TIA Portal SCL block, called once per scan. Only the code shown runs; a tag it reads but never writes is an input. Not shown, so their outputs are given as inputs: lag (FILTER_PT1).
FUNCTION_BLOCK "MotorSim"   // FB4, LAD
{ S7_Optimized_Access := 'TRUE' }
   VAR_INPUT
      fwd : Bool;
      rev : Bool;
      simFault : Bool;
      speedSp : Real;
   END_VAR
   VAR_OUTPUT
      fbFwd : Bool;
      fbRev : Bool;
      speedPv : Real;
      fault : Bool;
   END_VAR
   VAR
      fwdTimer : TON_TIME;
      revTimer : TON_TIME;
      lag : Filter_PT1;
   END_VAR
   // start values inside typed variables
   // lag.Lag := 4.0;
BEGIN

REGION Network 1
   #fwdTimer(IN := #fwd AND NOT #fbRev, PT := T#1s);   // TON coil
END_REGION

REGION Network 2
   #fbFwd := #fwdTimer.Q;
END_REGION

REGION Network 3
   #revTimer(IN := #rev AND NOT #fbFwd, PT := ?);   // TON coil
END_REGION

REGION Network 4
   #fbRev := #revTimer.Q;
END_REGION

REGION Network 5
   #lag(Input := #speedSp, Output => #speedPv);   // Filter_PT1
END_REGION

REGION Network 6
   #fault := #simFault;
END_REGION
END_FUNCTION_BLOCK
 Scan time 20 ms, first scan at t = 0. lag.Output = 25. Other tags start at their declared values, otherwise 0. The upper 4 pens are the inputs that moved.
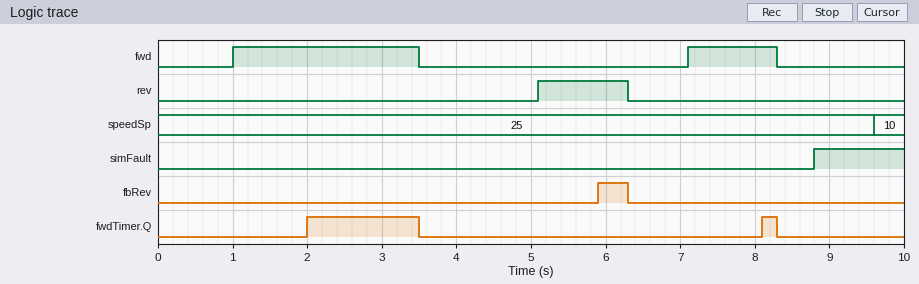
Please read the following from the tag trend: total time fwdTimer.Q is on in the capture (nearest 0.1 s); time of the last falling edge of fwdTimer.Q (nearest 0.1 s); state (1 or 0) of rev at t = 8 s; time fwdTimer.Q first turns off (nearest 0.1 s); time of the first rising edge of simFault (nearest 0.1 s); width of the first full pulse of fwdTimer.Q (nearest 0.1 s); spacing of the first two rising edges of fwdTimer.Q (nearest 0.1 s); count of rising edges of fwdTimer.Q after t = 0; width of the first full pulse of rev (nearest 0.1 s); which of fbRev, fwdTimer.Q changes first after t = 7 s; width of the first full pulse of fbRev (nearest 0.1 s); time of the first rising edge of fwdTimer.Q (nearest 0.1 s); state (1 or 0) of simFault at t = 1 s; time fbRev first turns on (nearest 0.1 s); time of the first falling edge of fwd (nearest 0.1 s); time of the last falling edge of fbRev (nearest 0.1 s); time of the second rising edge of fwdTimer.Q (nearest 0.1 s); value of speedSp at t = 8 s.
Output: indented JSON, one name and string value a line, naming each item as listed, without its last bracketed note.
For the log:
{
  "total time fwdTimer.Q is on in the capture": "1.7 s",
  "time of the last falling edge of fwdTimer.Q": "8.3 s",
  "state (1 or 0) of rev at t = 8 s": "0",
  "time fwdTimer.Q first turns off": "3.5 s",
  "time of the first rising edge of simFault": "8.8 s",
  "width of the first full pulse of fwdTimer.Q": "1.5 s",
  "spacing of the first two rising edges of fwdTimer.Q": "6.1 s",
  "count of rising edges of fwdTimer.Q after t = 0": "2",
  "width of the first full pulse of rev": "1.2 s",
  "which of fbRev, fwdTimer.Q changes first after t = 7 s": "fwdTimer.Q",
  "width of the first full pulse of fbRev": "0.4 s",
  "time of the first rising edge of fwdTimer.Q": "2.0 s",
  "state (1 or 0) of simFault at t = 1 s": "0",
  "time fbRev first turns on": "5.9 s",
  "time of the first falling edge of fwd": "3.5 s",
  "time of the last falling edge of fbRev": "6.3 s",
  "time of the second rising edge of fwdTimer.Q": "8.1 s",
  "value of speedSp at t = 8 s": "25"
}
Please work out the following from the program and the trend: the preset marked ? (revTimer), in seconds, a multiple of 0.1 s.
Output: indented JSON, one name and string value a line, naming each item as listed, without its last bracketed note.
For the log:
{
  "the preset marked ? (revTimer), in seconds, a multiple of 0.1 s": "0.8 s"
}
